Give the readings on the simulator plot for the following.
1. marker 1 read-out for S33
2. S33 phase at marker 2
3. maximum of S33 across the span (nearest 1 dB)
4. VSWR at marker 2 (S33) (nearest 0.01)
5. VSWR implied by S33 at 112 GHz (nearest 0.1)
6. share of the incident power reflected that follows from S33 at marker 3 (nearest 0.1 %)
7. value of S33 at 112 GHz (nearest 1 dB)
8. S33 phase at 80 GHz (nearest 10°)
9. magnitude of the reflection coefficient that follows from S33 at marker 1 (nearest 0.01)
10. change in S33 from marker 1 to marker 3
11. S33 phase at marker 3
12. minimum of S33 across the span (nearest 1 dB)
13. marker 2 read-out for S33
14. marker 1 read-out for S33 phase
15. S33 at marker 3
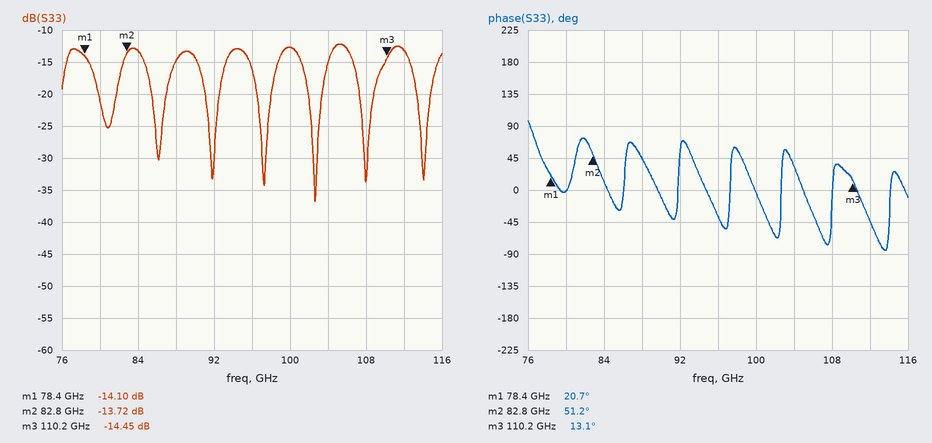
-14.10 dB
51.2°
-12 dB
1.52
1.6
3.6 %
-13 dB
0°
0.20
-0.35 dB
13.1°
-37 dB
-13.72 dB
20.7°
-14.45 dB
